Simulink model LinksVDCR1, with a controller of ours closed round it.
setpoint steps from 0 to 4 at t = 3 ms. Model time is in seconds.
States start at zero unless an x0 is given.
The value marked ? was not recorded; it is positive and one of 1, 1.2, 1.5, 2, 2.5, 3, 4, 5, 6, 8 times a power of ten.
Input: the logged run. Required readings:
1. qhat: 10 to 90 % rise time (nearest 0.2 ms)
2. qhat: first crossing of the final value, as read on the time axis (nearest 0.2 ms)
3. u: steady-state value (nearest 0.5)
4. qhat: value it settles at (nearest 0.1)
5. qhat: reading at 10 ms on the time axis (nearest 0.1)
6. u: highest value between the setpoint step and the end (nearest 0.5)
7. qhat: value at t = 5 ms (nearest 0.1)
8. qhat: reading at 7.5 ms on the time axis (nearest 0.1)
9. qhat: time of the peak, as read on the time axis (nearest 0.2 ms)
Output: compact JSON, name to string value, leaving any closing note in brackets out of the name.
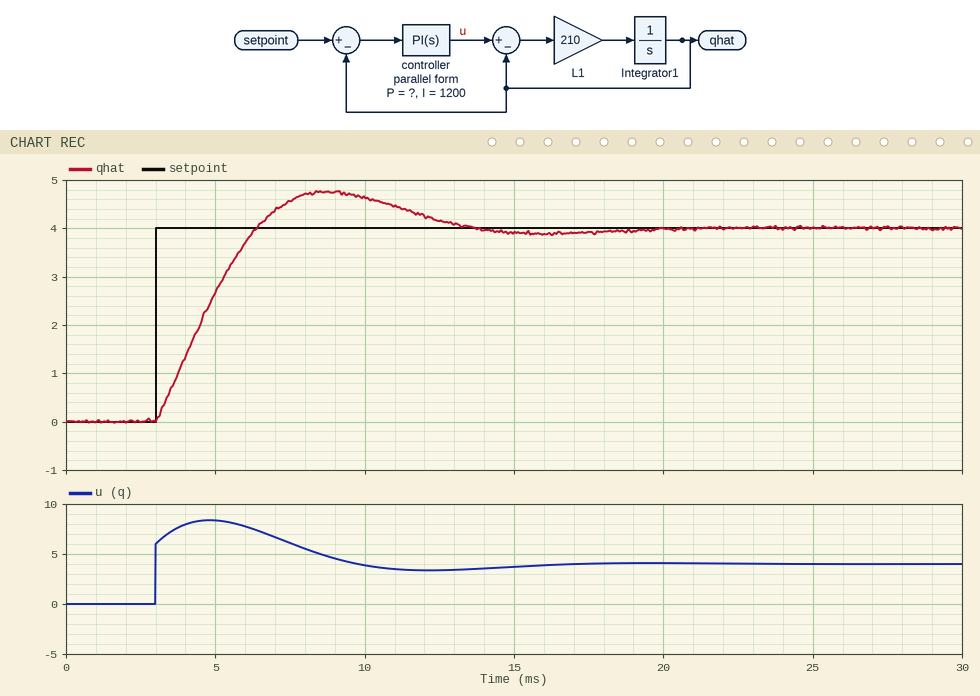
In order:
{"qhat: 10 to 90 % rise time": "2.6 ms", "qhat: first crossing of the final value, as read on the time axis": "6.4 ms", "u: steady-state value": "4.0", "qhat: value it settles at": "4.0", "qhat: reading at 10 ms on the time axis": "4.6", "u: highest value between the setpoint step and the end": "8.5", "qhat: value at t = 5 ms": "2.7", "qhat: reading at 7.5 ms on the time axis": "4.6", "qhat: time of the peak, as read on the time axis": "8.8 ms"}
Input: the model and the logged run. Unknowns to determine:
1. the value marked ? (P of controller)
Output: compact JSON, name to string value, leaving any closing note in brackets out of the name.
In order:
{"the value marked ?": "1.5"}
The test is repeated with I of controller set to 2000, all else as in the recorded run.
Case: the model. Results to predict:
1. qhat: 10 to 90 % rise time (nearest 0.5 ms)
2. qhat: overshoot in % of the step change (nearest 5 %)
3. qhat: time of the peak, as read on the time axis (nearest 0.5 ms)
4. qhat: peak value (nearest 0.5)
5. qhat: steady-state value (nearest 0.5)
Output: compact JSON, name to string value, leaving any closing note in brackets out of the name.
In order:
{"qhat: 10 to 90 % rise time": "2.0 ms", "qhat: overshoot in % of the step change": "30 %", "qhat: time of the peak, as read on the time axis": "7.5 ms", "qhat: peak value": "5.0", "qhat: steady-state value": "4.0"}
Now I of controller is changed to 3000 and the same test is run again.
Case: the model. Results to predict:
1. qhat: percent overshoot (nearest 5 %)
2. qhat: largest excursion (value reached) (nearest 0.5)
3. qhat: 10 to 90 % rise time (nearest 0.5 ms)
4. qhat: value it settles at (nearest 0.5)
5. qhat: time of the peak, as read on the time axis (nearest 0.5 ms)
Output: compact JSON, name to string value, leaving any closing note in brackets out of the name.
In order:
{"qhat: percent overshoot": "35 %", "qhat: largest excursion (value reached)": "5.5", "qhat: 10 to 90 % rise time": "1.5 ms", "qhat: value it settles at": "4.0", "qhat: time of the peak, as read on the time axis": "6.5 ms"}
